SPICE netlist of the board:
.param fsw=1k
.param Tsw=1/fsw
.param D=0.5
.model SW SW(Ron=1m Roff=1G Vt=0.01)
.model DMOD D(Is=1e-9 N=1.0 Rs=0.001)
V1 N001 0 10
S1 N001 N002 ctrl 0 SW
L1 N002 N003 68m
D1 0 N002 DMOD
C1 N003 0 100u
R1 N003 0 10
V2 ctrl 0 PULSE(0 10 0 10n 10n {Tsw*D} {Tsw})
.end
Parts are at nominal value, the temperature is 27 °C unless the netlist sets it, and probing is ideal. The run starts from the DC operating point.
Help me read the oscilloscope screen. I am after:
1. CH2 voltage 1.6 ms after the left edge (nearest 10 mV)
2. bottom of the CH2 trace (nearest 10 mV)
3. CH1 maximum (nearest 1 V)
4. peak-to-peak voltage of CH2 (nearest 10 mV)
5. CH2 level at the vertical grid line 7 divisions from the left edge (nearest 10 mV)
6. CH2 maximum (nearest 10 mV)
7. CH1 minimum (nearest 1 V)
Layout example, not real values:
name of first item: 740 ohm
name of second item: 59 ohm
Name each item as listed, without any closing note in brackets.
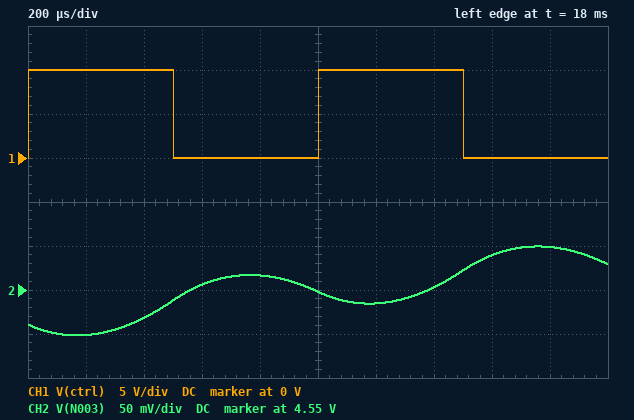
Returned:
CH2 voltage 1.6 ms after the left edge: 4.59 V
bottom of the CH2 trace: 4.50 V
CH1 maximum: 10 V
peak-to-peak voltage of CH2: 100 mV
CH2 level at the vertical grid line 7 divisions from the left edge: 4.55 V
CH2 maximum: 4.60 V
CH1 minimum: 0 V
